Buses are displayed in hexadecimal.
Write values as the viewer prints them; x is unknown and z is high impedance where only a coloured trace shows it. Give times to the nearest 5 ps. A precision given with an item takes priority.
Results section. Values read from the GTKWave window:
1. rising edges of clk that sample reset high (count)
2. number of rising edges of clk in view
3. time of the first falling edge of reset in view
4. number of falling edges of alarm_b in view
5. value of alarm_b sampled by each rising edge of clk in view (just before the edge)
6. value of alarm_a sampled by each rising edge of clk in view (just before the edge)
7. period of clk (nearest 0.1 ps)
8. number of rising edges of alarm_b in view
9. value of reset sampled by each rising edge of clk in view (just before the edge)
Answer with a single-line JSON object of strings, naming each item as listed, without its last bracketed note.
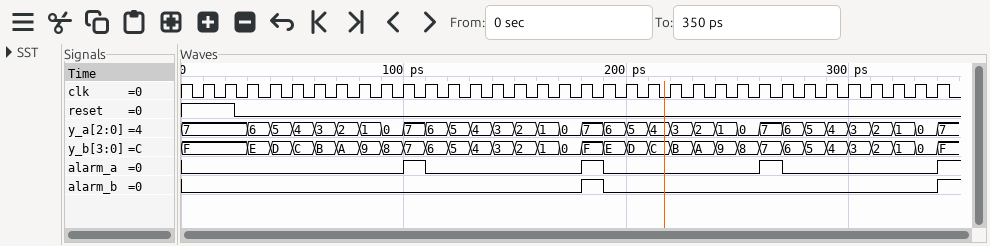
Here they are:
{"rising edges of clk that sample reset high": "2", "number of rising edges of clk in view": "34", "time of the first falling edge of reset in view": "25 ps", "number of falling edges of alarm_b in view": "1", "value of alarm_b sampled by each rising edge of clk in view": "0 0 0 0 0 0 0 0 0 0 0 0 0 0 0 0 0 0 1 0 0 0 0 0 0 0 0 0 0 0 0 0 0 0", "value of alarm_a sampled by each rising edge of clk in view": "0 0 0 0 0 0 0 0 0 0 1 0 0 0 0 0 0 0 1 0 0 0 0 0 0 0 1 0 0 0 0 0 0 0", "period of clk": "10 ps", "number of rising edges of alarm_b in view": "2", "value of reset sampled by each rising edge of clk in view": "1 1 0 0 0 0 0 0 0 0 0 0 0 0 0 0 0 0 0 0 0 0 0 0 0 0 0 0 0 0 0 0 0 0"}
